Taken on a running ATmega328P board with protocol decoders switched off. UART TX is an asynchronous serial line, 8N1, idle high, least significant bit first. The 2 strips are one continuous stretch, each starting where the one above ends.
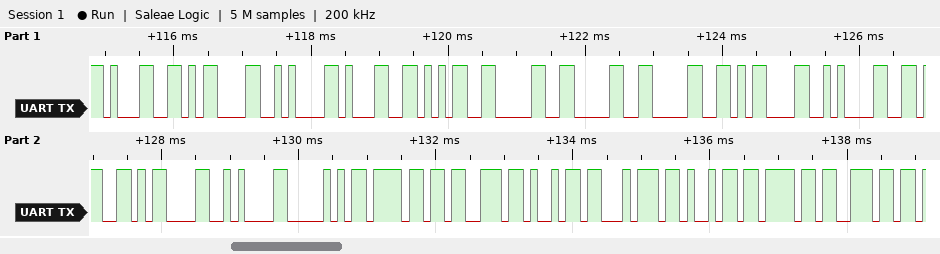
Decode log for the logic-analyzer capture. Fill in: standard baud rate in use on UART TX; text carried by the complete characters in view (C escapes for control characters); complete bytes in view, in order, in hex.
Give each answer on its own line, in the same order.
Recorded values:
9600 baud
"1\r\n15000\r\n6\r\nPosition"
31 0D 0A 31 35 30 30 30 0D 0A 36 0D 0A 50 6F 73 69 74 69 6F 6E
